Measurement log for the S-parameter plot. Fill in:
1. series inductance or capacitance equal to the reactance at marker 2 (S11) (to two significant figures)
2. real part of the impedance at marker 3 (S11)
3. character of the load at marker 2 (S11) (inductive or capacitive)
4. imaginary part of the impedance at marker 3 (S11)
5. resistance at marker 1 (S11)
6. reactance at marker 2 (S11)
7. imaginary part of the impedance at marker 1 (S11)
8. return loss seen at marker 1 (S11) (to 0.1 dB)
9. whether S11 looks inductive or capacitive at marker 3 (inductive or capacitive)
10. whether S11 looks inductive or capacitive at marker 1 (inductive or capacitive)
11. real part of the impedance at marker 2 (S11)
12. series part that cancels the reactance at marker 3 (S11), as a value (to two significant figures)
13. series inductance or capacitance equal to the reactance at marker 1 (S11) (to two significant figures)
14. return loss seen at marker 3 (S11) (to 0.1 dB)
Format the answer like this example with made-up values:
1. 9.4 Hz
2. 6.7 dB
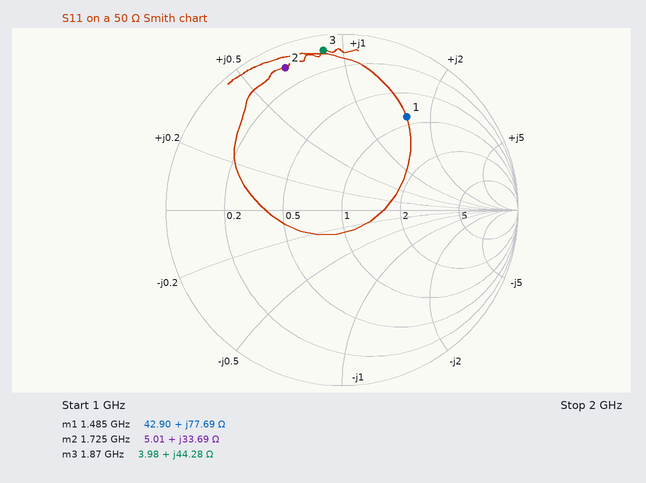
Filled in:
1. 3.1 nH
2. 3.98 Ω
3. inductive
4. +44.28 Ω
5. 42.90 Ω
6. +33.69 Ω
7. +77.69 Ω
8. 3.8 dB
9. inductive
10. inductive
11. 5.01 Ω
12. 1.9 pF
13. 8.3 nH
14. 0.8 dB
